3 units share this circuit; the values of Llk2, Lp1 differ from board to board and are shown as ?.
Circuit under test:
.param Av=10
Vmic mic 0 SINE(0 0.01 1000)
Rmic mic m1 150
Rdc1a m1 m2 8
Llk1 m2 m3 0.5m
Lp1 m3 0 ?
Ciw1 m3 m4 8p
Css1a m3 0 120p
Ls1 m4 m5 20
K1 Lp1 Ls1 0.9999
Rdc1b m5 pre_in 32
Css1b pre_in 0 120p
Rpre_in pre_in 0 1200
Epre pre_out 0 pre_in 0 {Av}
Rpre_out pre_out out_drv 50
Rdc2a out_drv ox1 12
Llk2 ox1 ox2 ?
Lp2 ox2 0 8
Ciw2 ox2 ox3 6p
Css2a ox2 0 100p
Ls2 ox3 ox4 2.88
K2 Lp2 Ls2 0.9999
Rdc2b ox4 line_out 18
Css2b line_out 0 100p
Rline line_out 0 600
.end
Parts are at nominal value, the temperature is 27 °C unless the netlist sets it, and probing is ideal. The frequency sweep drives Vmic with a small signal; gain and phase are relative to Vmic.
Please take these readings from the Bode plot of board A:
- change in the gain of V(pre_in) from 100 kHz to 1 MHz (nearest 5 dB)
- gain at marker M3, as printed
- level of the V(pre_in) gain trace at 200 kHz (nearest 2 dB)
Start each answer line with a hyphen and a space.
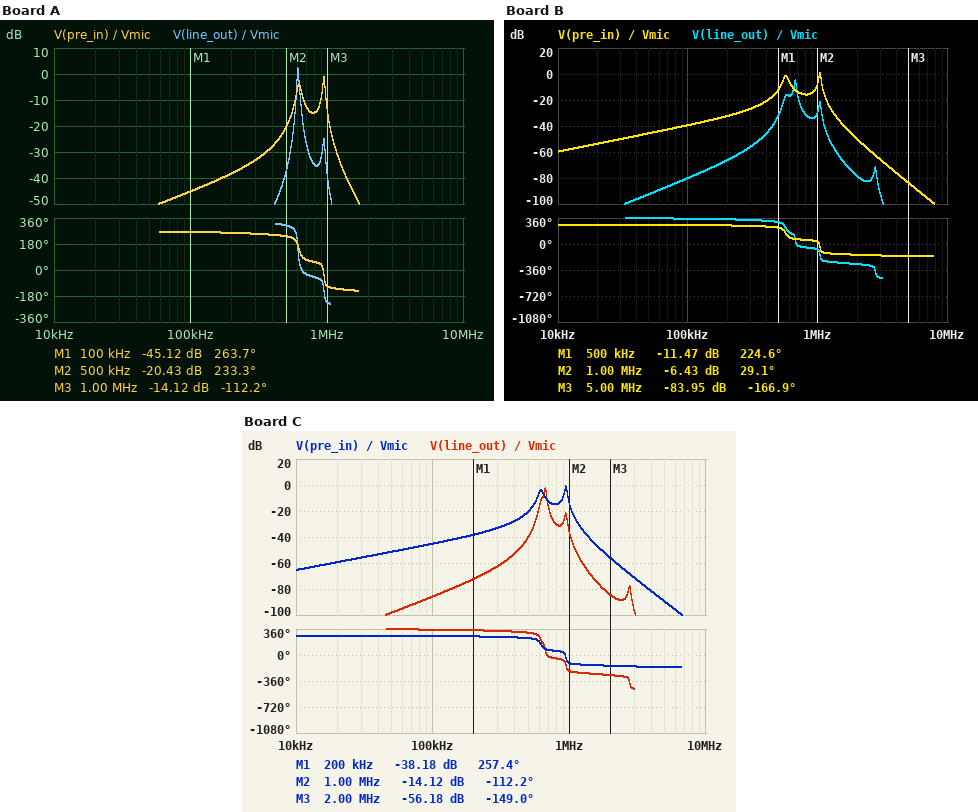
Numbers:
- 30 dB
- -14.12 dB
- -38 dB
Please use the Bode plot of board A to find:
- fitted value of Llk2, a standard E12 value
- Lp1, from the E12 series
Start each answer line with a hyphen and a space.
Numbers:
- 680 µH
- 5.6 H
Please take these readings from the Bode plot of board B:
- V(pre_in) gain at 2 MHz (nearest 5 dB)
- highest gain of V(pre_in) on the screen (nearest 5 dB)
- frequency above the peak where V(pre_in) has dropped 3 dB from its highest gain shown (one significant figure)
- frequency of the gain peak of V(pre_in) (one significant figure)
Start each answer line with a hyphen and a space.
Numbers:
- -50 dB
- 0 dB
- 1 MHz
- 1 MHz
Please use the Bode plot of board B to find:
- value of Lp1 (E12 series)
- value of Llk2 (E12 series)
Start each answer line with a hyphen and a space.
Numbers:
- 2.7 H
- 560 µH
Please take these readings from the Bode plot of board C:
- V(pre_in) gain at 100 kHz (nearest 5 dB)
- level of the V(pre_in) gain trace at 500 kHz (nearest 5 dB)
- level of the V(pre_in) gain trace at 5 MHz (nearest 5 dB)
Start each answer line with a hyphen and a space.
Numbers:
- -45 dB
- -20 dB
- -90 dB
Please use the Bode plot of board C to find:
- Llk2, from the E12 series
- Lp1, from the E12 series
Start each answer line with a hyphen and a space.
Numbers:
- 560 µH
- 5.6 H
